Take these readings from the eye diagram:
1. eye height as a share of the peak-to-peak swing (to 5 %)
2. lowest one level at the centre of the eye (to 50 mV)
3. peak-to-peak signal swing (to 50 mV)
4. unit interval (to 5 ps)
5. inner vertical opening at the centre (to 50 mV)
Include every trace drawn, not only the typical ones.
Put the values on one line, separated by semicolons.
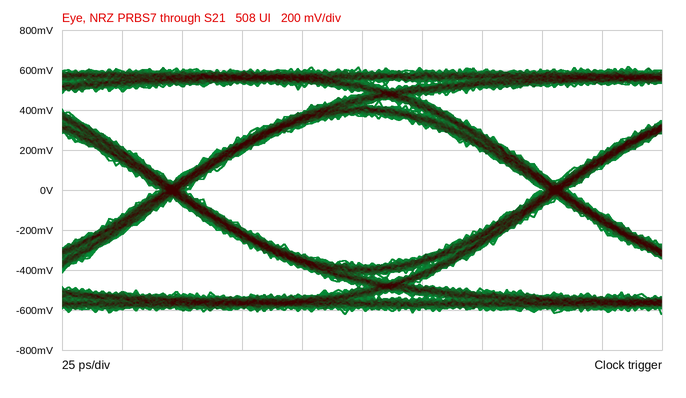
60 %; 350 mV; 1.25 V; 160 ps; 750 mV
